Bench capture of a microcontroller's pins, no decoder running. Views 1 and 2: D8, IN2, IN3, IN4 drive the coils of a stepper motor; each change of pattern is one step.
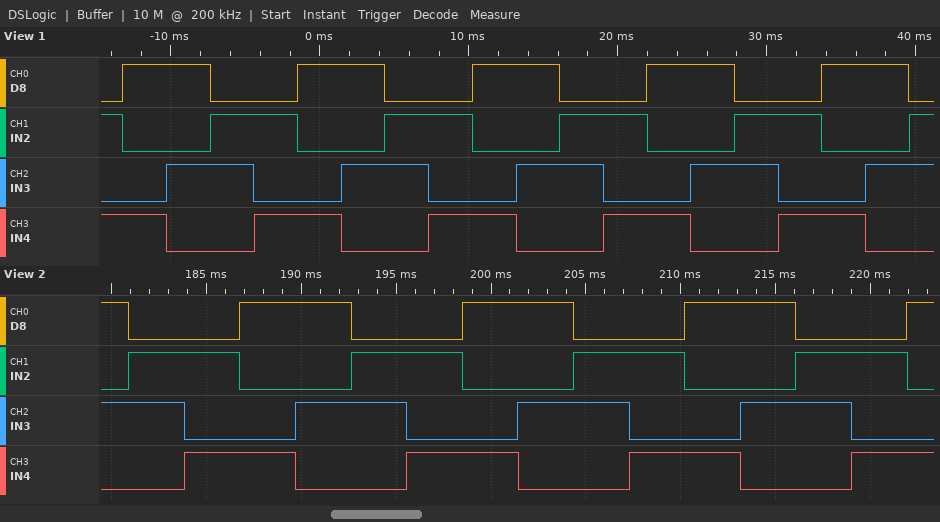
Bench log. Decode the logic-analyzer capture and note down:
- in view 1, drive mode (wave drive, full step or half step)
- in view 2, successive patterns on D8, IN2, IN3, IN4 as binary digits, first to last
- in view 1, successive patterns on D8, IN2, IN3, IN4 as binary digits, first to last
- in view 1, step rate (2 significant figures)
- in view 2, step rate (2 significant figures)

full step
1010 0110 0101 1001 1010 0110 0101 1001 1010 0110 0101 1001 1010 0110 0101 1001
0101 1001 1010 0110 0101 1001 1010 0110 0101 1001 1010 0110 0101 1001 1010 0110 0101 1001 1010 0110
340 steps/s
340 steps/s
